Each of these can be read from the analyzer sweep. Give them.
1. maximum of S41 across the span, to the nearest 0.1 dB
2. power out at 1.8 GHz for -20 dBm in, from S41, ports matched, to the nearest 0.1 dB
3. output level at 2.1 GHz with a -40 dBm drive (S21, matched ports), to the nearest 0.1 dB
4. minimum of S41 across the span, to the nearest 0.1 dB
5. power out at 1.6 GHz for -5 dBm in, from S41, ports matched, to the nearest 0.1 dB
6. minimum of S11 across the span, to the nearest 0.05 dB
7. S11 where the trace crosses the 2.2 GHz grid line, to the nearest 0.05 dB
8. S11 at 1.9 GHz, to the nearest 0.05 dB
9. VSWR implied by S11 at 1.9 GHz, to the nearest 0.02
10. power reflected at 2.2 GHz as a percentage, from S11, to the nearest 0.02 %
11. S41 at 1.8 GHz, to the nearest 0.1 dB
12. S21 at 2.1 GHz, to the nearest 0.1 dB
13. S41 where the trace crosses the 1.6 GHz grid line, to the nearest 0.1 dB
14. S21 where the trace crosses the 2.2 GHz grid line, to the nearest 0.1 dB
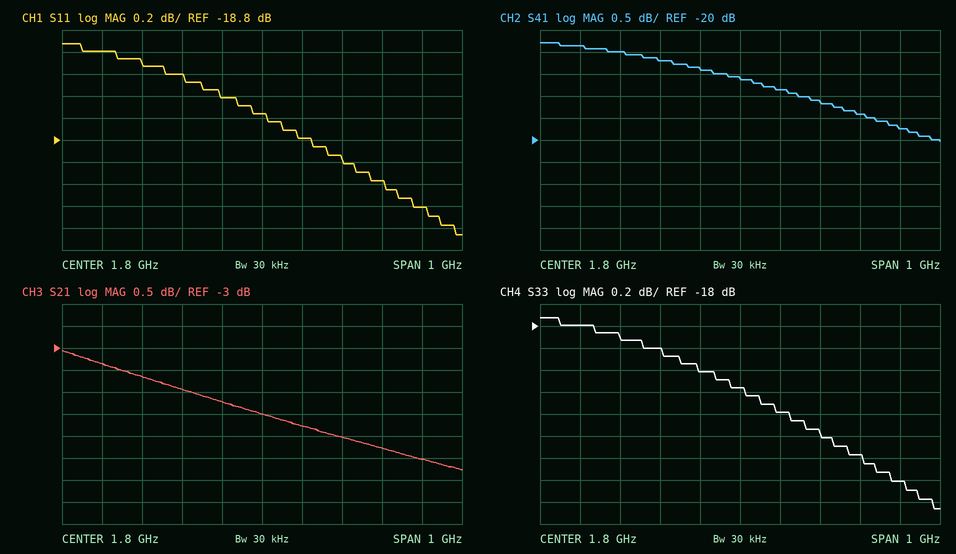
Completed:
-17.8 dB
-38.6 dBm
-45.3 dBm
-20.0 dB
-23.2 dBm
-19.65 dB
-19.40 dB
-18.80 dB
1.26
1.14 %
-18.6 dB
-5.3 dB
-18.2 dB
-5.5 dB
